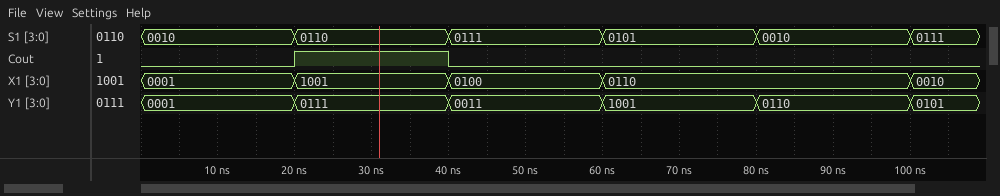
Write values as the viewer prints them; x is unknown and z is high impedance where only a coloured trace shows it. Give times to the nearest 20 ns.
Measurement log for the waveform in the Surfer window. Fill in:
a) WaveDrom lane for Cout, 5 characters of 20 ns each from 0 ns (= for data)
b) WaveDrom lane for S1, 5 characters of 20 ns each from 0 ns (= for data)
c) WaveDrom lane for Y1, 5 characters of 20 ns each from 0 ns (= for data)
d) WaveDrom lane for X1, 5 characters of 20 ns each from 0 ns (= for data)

{name: 'Cout', wave: '010..'}
{name: 'S1', wave: '=====', data: '0010 0110 0111 0101 0010'}
{name: 'Y1', wave: '=====', data: '0001 0111 0011 1001 0110'}
{name: 'X1', wave: '====.', data: '0001 1001 0100 0110'}
